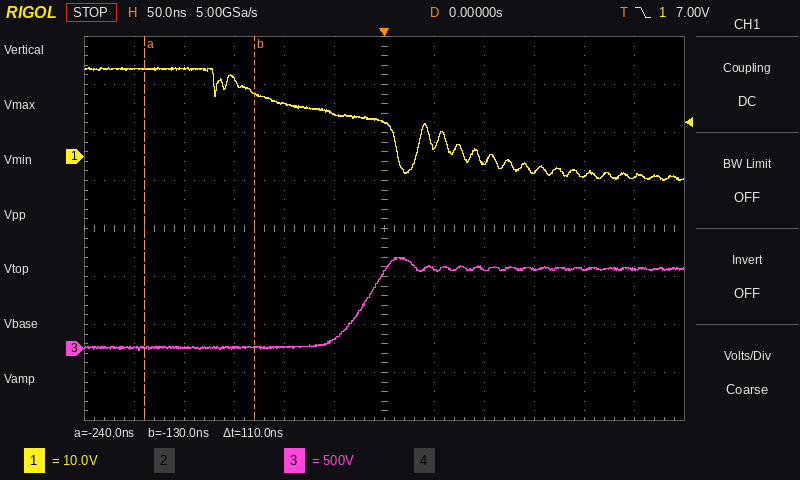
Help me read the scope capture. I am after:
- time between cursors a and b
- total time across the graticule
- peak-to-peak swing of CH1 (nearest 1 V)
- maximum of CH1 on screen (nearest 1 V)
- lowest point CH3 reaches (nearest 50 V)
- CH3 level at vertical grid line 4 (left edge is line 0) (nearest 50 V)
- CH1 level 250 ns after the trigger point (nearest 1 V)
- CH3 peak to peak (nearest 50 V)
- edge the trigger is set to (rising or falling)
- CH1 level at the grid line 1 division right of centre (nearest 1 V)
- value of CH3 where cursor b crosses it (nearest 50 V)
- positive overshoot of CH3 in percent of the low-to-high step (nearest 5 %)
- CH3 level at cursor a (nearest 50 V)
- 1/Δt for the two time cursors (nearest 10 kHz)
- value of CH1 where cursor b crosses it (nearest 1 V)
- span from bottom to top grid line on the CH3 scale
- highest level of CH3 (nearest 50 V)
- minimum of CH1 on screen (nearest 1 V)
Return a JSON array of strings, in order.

["110 ns", "600 ns", "24 V", "19 V", "0 V", "0 V", "-4 V", "950 V", "falling", "2 V", "0 V", "15 %", "0 V", "9.09 MHz", "13 V", "4 kV", "950 V", "-5 V"]
